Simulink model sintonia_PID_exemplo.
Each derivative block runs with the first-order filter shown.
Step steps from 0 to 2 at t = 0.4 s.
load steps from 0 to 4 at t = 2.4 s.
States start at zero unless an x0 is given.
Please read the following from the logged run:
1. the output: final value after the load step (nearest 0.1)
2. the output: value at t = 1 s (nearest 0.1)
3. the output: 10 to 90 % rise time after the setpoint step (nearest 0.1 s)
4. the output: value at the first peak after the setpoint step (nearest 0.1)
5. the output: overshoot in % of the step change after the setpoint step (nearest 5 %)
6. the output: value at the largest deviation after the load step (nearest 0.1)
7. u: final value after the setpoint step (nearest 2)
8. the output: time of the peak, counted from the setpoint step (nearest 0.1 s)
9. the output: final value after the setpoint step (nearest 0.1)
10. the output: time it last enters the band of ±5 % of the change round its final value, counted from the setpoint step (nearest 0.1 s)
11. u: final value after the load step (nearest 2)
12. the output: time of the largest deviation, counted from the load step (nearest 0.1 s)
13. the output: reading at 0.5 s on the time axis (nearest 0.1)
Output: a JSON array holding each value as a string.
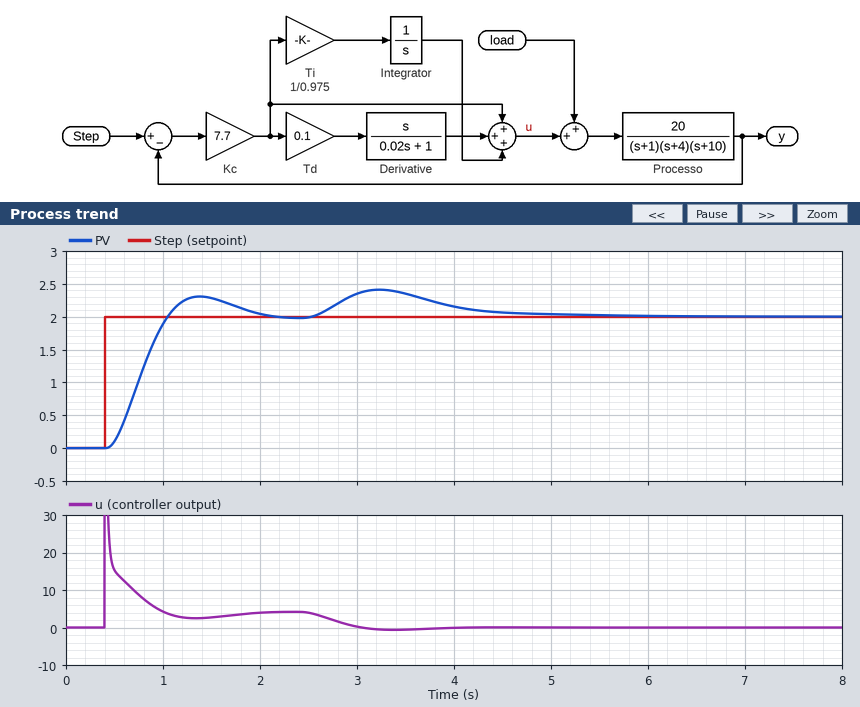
["2.0", "1.9", "0.4 s", "2.3", "15 %", "2.4", "4", "1.0 s", "2.0", "1.5 s", "0", "0.8 s", "0.1"]
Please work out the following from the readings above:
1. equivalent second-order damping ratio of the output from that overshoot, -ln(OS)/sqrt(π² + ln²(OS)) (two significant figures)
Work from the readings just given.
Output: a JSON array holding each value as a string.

["0.52"]
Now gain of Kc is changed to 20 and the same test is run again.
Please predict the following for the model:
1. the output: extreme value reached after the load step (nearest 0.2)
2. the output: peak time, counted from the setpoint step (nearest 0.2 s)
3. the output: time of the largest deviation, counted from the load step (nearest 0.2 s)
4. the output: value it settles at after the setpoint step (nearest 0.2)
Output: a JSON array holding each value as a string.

["2.2", "0.6 s", "0.6 s", "2.0"]
